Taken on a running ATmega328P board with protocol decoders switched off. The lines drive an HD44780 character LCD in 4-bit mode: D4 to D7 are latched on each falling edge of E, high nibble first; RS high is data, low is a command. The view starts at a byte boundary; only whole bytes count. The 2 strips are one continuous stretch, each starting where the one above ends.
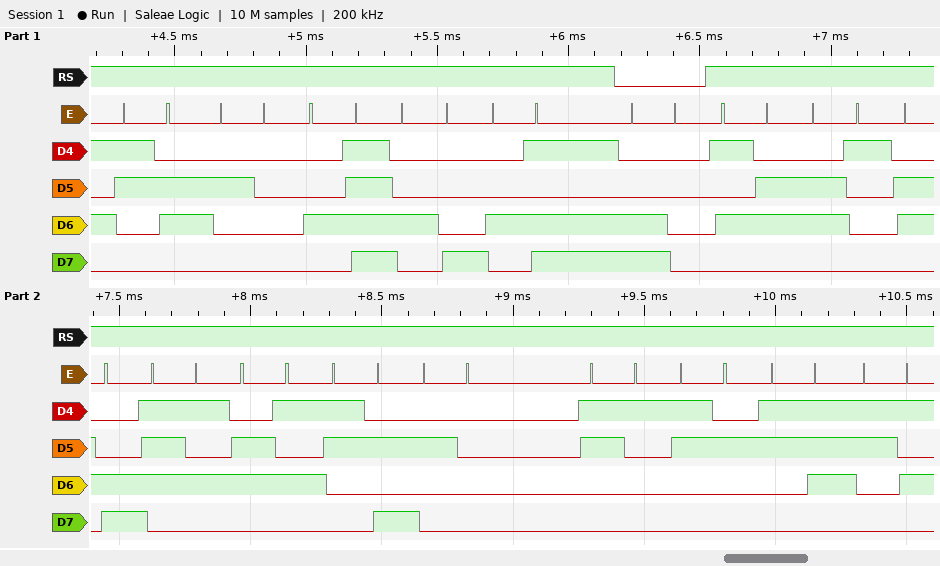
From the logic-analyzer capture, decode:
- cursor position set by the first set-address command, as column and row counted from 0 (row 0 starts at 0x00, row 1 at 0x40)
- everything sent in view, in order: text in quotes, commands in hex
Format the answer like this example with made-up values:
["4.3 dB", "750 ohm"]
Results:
["column 0, row 1", "\"6 OHM\" 0xC0 \"Value: 1275\""]
